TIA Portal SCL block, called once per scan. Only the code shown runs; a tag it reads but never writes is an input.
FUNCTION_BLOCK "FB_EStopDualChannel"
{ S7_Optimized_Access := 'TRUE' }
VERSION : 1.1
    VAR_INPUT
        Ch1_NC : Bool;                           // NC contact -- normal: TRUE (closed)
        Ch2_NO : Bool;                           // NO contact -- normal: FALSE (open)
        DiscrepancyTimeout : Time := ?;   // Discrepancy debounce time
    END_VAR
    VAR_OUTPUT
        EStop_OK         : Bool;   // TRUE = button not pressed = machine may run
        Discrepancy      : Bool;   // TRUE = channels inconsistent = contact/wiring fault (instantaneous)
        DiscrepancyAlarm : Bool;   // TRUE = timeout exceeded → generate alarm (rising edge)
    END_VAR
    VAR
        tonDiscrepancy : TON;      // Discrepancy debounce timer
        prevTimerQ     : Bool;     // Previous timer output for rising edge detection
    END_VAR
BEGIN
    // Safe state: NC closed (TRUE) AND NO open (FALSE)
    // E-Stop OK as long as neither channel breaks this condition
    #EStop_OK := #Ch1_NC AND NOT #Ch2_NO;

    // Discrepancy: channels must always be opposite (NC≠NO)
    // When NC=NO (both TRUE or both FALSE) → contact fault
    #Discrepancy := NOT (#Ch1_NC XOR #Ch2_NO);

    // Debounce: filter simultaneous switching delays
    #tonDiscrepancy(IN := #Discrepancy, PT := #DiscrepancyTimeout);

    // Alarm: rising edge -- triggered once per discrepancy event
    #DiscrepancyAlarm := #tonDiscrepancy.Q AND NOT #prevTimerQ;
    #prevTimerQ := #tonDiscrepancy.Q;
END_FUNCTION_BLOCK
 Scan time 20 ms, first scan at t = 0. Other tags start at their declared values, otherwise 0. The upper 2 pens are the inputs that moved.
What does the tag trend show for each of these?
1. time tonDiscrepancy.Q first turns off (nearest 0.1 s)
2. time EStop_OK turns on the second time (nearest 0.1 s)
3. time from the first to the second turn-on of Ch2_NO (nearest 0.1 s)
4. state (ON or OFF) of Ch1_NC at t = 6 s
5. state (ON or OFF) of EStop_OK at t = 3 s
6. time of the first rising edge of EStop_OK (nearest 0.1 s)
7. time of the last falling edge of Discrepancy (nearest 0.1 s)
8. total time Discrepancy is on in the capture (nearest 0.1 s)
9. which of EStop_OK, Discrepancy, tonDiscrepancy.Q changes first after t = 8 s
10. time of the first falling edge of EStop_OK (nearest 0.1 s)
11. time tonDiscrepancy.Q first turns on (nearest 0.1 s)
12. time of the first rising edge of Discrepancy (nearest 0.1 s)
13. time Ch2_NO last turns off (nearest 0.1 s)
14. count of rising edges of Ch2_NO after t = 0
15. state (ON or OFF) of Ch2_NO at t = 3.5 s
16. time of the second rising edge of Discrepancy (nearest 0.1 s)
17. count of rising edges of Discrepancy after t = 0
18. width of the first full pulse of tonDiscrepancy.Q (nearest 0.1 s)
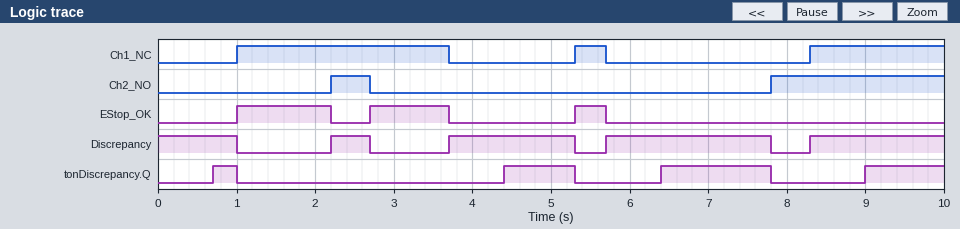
1.0 s
2.7 s
5.6 s
OFF
ON
1.0 s
7.8 s
6.9 s
Discrepancy
2.2 s
0.7 s
2.2 s
2.7 s
2
OFF
3.7 s
4
0.3 s
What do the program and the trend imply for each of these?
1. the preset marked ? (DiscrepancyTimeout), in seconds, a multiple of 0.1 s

0.7 s
